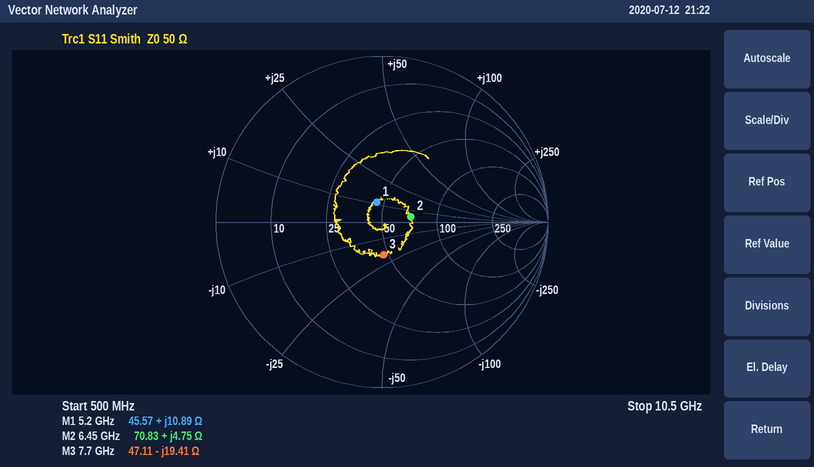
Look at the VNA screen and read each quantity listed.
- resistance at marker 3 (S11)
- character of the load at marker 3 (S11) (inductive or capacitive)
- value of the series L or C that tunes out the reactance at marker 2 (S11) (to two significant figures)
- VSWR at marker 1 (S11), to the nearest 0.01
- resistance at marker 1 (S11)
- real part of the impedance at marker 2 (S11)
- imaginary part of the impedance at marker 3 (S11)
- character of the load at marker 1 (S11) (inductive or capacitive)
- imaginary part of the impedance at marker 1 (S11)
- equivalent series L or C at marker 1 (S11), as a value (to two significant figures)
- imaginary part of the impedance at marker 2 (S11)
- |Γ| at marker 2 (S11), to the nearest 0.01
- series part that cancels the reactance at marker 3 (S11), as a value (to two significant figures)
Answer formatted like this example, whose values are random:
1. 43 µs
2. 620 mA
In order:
1. 47.11 Ω
2. capacitive
3. 5.2 pF
4. 1.28
5. 45.57 Ω
6. 70.83 Ω
7. -19.41 Ω
8. inductive
9. +10.89 Ω
10. 330 pH
11. +4.75 Ω
12. 0.18
13. 400 pH
